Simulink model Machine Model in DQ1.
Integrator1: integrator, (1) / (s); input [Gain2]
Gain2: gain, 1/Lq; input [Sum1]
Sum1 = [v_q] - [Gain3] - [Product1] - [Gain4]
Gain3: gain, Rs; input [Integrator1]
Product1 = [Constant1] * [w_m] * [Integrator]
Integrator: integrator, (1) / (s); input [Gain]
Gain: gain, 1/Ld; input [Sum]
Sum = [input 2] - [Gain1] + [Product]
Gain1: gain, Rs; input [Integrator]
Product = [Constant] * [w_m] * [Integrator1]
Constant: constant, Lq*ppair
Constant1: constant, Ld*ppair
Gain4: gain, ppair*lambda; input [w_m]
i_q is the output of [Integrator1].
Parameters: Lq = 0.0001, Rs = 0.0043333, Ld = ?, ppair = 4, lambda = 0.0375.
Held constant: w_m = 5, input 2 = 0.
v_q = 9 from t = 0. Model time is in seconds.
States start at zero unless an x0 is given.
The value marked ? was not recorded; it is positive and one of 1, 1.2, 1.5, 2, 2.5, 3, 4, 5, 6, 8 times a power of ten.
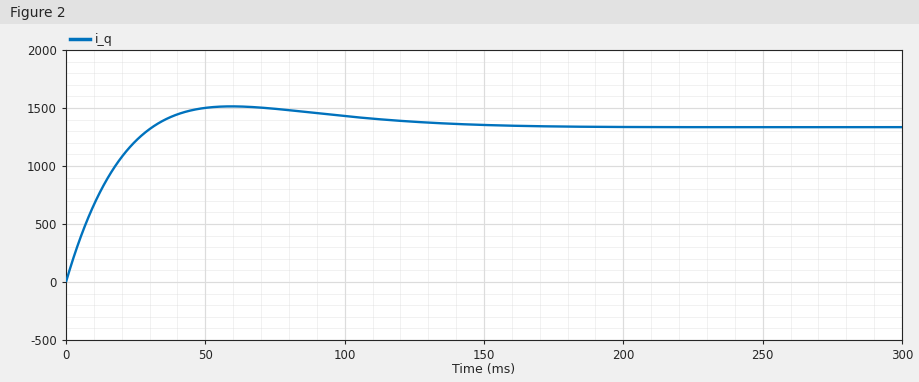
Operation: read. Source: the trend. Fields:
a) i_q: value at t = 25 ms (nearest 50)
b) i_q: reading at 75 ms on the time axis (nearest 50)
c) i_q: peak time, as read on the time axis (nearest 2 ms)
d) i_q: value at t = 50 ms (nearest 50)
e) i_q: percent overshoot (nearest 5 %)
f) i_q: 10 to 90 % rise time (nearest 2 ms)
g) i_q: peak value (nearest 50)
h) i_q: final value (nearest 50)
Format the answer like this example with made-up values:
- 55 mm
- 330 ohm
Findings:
- 1200
- 1500
- 60 ms
- 1500
- 15 %
- 22 ms
- 1500
- 1350
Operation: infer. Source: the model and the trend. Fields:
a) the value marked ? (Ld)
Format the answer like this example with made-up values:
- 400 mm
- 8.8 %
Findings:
- 0.0002
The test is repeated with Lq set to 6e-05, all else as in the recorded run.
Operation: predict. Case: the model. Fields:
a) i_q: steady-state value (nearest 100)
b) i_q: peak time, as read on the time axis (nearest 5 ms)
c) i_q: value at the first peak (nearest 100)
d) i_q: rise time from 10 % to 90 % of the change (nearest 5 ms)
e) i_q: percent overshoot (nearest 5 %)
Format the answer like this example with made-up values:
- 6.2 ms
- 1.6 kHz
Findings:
- 1500
- 45 ms
- 1700
- 15 ms
- 10 %
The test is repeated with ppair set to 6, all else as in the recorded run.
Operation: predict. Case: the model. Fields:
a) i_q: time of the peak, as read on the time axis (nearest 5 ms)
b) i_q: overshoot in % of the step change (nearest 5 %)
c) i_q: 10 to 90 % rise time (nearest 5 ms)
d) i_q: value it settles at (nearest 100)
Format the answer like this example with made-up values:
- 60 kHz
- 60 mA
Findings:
- 45 ms
- 35 %
- 15 ms
- 900
